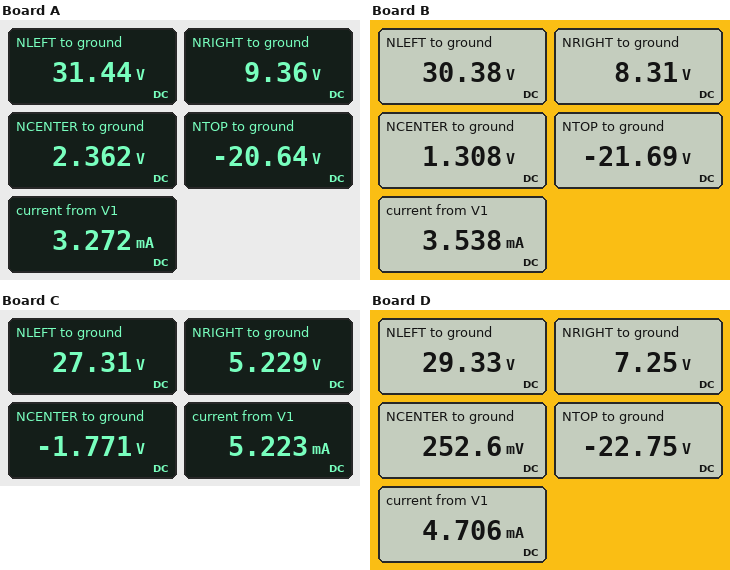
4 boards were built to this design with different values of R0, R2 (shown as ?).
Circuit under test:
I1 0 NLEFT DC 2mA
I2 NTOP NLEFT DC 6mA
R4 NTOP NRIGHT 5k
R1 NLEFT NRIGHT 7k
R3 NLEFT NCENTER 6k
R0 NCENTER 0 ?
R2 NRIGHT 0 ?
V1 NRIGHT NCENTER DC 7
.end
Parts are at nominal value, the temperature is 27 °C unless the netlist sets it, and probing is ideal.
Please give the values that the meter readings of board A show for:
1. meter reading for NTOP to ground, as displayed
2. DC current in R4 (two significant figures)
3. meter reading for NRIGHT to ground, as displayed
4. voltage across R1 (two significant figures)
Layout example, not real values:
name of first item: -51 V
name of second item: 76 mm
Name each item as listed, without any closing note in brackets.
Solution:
meter reading for NTOP to ground, as displayed: -20.64 V
DC current in R4: 6.0 mA
meter reading for NRIGHT to ground, as displayed: 9.36 V
voltage across R1: 22 V
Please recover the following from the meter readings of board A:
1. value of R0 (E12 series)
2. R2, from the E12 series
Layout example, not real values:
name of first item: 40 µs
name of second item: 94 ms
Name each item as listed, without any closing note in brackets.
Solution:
value of R0: 1.5 kΩ
R2, from the E12 series: 22 kΩ
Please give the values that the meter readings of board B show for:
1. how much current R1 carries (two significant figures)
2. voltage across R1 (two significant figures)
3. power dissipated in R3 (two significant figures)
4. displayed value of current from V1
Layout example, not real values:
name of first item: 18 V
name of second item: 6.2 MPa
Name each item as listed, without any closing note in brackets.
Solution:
how much current R1 carries: 3.2 mA
voltage across R1: 22 V
power dissipated in R3: 140 mW
displayed value of current from V1: 3.538 mA
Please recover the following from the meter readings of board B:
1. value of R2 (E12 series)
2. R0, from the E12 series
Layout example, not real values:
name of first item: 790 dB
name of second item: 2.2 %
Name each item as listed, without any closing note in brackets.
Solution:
value of R2: 12 kΩ
R0, from the E12 series: 1 kΩ
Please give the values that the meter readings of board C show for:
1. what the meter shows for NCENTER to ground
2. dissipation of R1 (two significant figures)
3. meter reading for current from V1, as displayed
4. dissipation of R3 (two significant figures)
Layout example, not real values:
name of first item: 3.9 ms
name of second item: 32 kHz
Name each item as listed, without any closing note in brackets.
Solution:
what the meter shows for NCENTER to ground: -1.771 V
dissipation of R1: 70 mW
meter reading for current from V1, as displayed: 5.223 mA
dissipation of R3: 140 mW
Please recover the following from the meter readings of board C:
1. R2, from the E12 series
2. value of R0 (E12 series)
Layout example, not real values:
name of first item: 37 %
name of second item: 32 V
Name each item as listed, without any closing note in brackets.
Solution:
R2, from the E12 series: 2.2 kΩ
value of R0: 4.7 kΩ
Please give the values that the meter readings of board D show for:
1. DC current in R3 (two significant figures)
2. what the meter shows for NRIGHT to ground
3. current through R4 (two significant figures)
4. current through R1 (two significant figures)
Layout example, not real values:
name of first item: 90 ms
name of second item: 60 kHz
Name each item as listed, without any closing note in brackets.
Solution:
DC current in R3: 4.8 mA
what the meter shows for NRIGHT to ground: 7.25 V
current through R4: 6.0 mA
current through R1: 3.2 mA
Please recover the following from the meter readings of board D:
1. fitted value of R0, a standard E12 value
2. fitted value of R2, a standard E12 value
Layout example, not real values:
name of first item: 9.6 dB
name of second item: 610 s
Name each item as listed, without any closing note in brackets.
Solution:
fitted value of R0, a standard E12 value: 1.8 kΩ
fitted value of R2, a standard E12 value: 3.9 kΩ
